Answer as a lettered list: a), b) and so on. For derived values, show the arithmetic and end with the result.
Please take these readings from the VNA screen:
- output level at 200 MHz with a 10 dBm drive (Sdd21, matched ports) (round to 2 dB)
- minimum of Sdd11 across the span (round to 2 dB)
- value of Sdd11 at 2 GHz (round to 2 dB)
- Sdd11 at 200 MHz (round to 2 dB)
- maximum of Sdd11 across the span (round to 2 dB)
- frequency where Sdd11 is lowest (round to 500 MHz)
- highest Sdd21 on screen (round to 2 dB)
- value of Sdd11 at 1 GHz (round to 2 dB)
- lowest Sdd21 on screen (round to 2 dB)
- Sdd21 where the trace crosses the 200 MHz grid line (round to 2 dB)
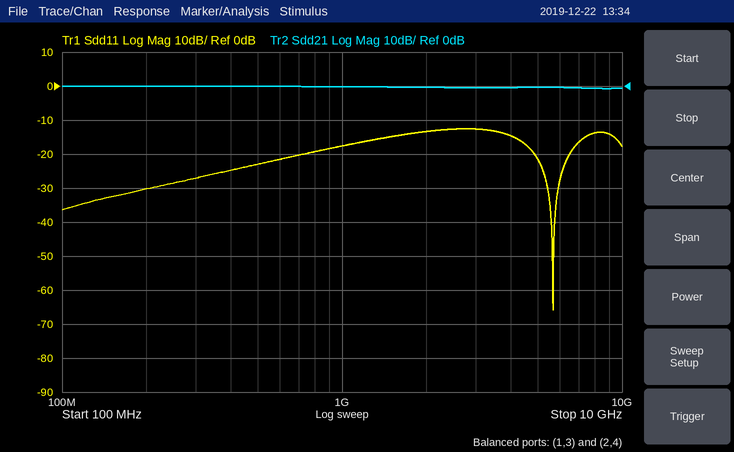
a) 10 dBm + (0 dB) = 10 dBm
b) -66 dB
c) -14 dB
d) -30 dB
e) -12 dB
f) 5.5 GHz
g) 0 dB
h) -18 dB
i) 0 dB
j) 0 dB
